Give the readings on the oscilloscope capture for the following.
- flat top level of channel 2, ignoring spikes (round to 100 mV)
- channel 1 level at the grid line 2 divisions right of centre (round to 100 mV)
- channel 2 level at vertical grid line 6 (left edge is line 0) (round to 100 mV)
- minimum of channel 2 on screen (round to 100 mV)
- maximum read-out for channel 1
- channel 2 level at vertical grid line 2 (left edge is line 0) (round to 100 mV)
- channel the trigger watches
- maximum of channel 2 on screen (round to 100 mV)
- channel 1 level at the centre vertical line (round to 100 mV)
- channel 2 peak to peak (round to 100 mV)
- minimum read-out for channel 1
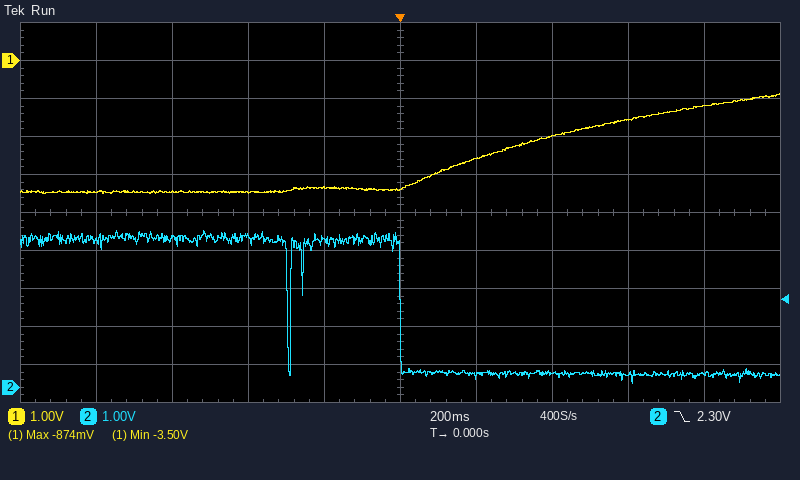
3.9 V
-2.0 V
300 mV
100 mV
-874 mV
3.9 V
channel 2
4.1 V
-3.4 V
4.0 V
-3.50 V
